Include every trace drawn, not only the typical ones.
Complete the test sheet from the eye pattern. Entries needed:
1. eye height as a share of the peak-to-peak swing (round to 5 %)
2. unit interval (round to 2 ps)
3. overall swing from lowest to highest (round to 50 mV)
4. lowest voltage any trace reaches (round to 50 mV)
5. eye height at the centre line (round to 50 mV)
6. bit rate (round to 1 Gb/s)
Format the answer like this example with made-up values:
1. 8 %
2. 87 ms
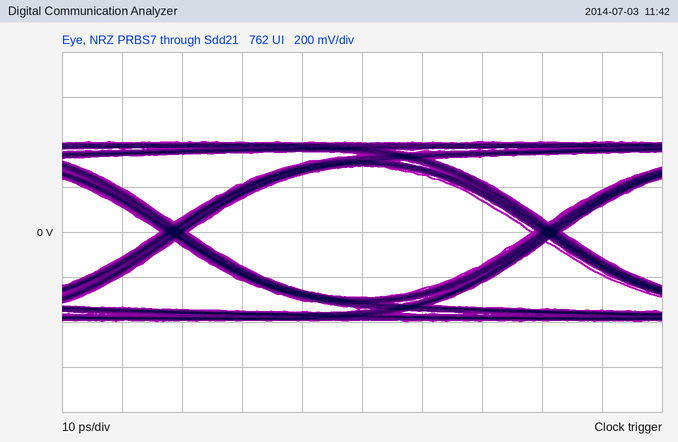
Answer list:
1. 75 %
2. 62 ps
3. 800 mV
4. -400 mV
5. 600 mV
6. 16 Gb/s
